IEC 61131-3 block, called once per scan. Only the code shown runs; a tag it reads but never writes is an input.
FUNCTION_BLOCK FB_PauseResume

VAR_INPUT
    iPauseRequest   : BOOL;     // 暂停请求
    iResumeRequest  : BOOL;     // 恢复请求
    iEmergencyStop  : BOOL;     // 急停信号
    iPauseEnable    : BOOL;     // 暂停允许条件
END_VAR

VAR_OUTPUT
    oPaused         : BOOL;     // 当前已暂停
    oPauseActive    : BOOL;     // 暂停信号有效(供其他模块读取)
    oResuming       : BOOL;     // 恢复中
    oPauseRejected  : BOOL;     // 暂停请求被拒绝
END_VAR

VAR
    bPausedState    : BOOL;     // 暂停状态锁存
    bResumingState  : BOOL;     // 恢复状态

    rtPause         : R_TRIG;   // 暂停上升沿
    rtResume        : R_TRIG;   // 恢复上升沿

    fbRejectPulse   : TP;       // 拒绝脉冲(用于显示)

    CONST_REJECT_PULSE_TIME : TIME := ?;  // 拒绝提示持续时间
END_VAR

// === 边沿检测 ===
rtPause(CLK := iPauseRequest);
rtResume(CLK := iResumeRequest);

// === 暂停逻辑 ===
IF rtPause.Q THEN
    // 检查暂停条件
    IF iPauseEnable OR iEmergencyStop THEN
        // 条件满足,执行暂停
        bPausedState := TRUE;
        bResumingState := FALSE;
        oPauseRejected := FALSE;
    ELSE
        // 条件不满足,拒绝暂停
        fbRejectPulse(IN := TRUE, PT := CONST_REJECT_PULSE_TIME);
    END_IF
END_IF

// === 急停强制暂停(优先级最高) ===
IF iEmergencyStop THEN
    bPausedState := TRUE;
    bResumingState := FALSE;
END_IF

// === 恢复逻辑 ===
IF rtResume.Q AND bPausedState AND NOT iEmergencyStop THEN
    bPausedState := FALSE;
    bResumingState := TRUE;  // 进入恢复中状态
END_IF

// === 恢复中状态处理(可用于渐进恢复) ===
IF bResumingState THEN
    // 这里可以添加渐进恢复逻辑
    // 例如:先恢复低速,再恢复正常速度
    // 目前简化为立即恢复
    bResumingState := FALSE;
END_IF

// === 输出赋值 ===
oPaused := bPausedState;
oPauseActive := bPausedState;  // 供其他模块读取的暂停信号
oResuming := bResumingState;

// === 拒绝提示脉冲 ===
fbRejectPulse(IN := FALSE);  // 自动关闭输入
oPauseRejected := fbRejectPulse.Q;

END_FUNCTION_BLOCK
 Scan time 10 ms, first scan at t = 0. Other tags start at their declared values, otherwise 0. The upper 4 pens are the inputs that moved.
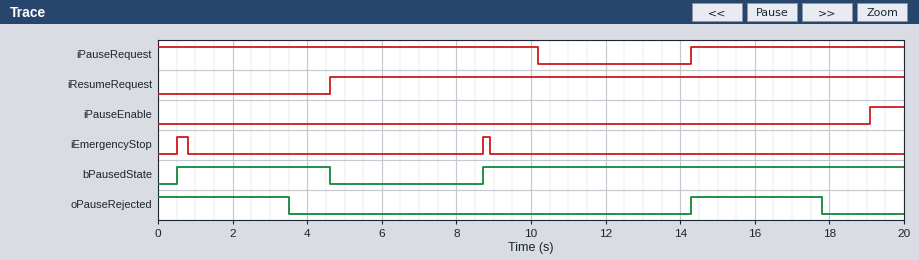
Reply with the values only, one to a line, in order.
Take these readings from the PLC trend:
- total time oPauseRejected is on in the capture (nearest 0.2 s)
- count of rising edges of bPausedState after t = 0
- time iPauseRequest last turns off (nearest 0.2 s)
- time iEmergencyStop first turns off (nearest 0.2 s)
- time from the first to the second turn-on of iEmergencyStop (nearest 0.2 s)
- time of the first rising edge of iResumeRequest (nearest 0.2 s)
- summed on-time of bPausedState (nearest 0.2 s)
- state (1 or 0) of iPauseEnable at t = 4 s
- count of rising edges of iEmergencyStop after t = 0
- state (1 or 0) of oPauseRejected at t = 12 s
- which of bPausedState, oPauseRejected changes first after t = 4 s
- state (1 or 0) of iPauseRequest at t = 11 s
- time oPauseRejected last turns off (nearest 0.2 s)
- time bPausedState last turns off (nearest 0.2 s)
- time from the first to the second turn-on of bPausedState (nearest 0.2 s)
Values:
7.0 s
2
10.2 s
0.8 s
8.2 s
4.6 s
15.4 s
0
2
0
bPausedState
0
17.8 s
4.6 s
8.2 s
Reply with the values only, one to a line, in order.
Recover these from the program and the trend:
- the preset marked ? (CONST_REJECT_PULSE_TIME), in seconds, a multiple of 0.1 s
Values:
3.5 s
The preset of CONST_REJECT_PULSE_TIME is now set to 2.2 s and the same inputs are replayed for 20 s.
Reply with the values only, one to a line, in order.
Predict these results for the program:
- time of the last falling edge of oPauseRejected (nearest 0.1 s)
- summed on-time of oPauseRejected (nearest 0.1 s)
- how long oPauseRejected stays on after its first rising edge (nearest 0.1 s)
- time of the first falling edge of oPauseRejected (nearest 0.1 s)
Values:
16.5 s
4.4 s
2.2 s
2.2 s
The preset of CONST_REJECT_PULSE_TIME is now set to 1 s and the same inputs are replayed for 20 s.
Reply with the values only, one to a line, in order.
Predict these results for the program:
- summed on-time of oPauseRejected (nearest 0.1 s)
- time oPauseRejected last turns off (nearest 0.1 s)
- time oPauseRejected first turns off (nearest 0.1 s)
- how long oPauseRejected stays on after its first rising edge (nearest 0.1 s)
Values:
2.0 s
15.3 s
1.0 s
1.0 s
